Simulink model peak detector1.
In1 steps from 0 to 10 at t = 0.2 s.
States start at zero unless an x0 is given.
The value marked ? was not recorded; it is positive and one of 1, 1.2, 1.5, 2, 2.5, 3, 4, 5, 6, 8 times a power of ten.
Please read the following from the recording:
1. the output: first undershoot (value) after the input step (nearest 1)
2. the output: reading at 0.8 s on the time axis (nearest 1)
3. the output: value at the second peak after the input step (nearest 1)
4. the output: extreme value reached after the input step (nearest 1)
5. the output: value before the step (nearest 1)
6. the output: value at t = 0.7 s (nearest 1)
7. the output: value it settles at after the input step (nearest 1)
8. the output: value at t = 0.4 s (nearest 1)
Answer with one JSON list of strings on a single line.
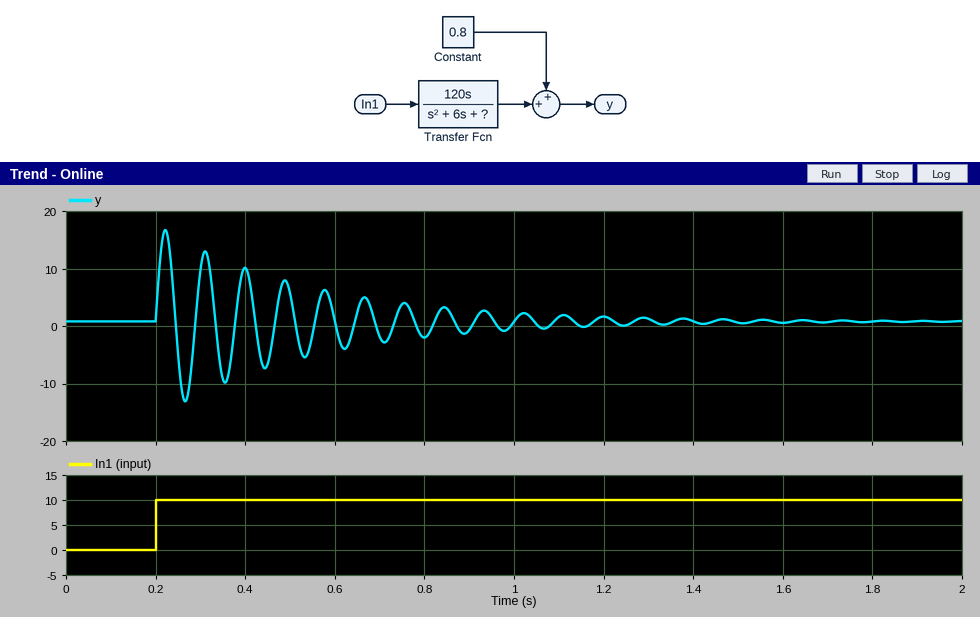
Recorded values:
["-13", "-2", "13", "17", "1", "-2", "1", "10"]
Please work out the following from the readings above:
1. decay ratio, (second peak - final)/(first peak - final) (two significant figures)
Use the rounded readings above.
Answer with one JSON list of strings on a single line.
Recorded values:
["0.75"]
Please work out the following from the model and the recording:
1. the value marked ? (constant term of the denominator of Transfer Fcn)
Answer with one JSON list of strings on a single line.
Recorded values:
["5000"]
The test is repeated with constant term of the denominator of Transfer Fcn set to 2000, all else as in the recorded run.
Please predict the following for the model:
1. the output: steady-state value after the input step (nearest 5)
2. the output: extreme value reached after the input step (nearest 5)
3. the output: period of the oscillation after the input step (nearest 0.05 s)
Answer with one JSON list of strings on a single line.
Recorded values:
["0", "25", "0.15 s"]
